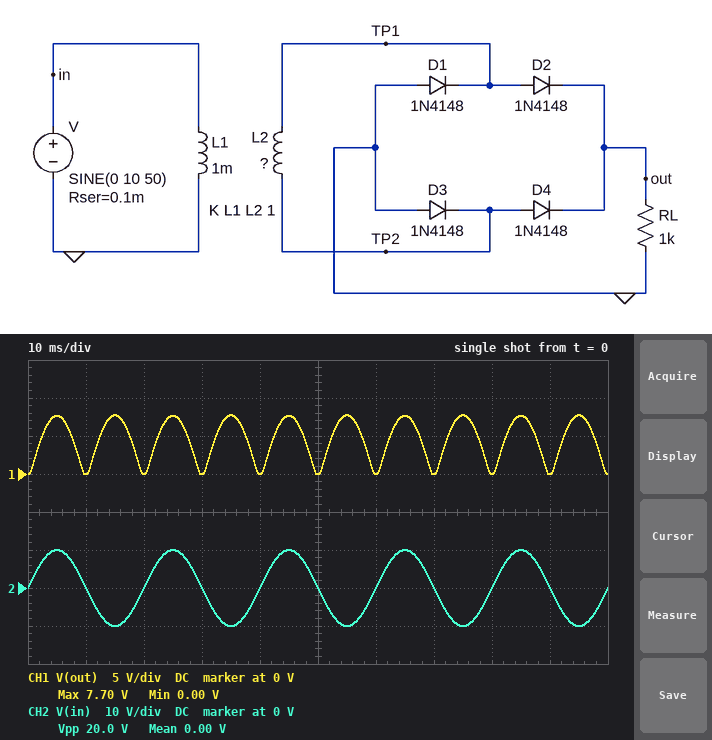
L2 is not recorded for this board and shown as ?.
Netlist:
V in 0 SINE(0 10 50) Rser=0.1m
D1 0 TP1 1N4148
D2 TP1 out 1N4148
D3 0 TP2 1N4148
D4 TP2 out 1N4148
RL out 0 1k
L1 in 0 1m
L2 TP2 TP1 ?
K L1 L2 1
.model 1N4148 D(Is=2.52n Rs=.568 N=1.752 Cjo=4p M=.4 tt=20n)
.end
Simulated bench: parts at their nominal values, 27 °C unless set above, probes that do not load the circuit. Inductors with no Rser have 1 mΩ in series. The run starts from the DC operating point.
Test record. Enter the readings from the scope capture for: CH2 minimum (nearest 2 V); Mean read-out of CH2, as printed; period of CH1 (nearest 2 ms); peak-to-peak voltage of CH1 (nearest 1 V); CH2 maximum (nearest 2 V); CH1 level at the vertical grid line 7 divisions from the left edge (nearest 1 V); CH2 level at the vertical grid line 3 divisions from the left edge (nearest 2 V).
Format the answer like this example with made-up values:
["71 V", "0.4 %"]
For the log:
["-10 V", "0.00 V", "10 ms", "8 V", "10 V", "0 V", "0 V"]
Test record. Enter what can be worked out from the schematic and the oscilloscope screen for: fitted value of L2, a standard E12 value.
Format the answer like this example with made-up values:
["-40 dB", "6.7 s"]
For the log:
["820 µH"]
